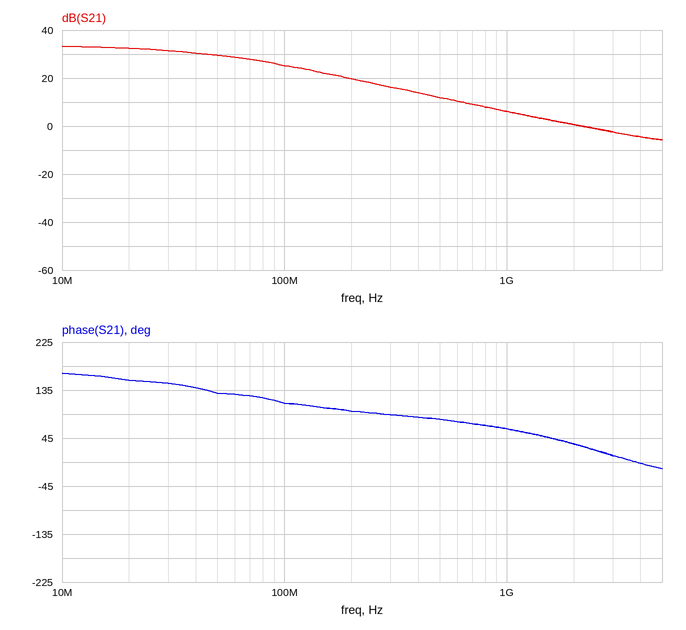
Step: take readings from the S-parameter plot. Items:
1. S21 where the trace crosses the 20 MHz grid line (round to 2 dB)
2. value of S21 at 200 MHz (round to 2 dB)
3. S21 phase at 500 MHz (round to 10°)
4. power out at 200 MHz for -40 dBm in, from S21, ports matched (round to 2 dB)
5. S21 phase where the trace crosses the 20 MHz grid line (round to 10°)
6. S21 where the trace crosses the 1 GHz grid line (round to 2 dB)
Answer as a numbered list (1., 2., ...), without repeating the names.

1. 32 dB
2. 20 dB
3. 80°
4. -20 dBm
5. 150°
6. 6 dB
